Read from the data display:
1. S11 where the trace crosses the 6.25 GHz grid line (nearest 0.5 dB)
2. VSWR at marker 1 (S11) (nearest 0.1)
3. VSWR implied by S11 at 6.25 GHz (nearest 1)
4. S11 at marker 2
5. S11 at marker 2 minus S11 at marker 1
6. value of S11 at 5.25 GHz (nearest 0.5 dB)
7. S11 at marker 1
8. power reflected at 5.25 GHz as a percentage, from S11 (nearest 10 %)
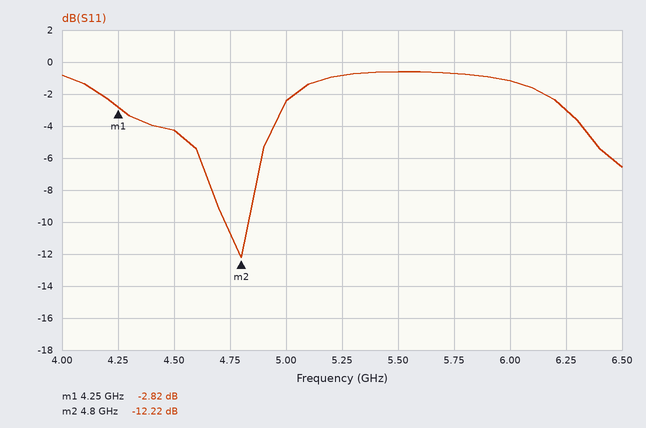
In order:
-3.0 dB
6.2
6
-12.22 dB
-9.40 dB
-1.0 dB
-2.82 dB
80 %
